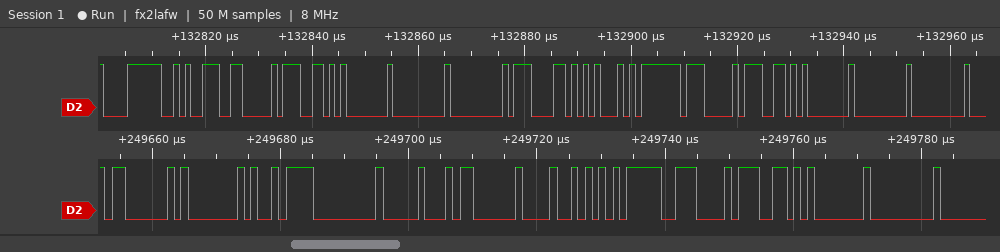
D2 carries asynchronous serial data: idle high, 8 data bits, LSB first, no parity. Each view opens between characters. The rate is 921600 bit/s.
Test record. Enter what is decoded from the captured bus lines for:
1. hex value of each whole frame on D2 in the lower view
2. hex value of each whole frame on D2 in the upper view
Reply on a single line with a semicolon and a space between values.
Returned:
03, 01, E9, 00, 10, 03, 48, F5, 0E, 67, 01, 00; F8, CA, 06, 67, 01, 00, 00, 87, 15, FD, 07, 67, 01, 00, 00
